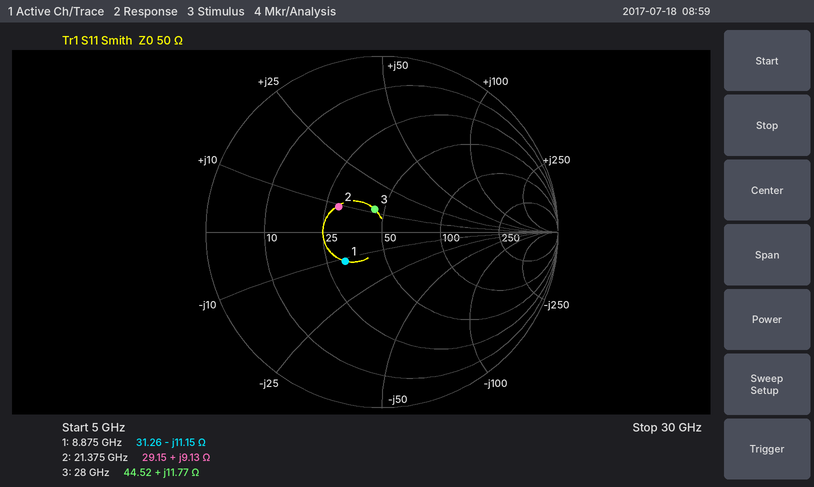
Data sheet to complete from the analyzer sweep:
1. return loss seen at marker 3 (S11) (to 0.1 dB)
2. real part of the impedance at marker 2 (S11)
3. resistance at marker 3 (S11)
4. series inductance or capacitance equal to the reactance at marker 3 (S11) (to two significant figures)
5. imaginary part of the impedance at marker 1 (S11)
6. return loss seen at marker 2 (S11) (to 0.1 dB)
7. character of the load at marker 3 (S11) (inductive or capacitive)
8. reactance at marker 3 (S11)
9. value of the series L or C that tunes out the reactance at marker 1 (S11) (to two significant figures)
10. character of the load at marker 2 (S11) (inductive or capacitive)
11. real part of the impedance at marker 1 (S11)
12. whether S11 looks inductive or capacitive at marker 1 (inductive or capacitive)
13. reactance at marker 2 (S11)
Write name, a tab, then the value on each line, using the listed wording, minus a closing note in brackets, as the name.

return loss seen at marker 3 (S11)	17.3 dB
real part of the impedance at marker 2	29.15 Ω
resistance at marker 3	44.52 Ω
series inductance or capacitance equal to the reactance at marker 3 (S11)	67 pH
imaginary part of the impedance at marker 1	-11.15 Ω
return loss seen at marker 2 (S11)	10.9 dB
character of the load at marker 3 (S11)	inductive
reactance at marker 3	+11.77 Ω
value of the series L or C that tunes out the reactance at marker 1 (S11)	200 pH
character of the load at marker 2 (S11)	inductive
real part of the impedance at marker 1	31.26 Ω
whether S11 looks inductive or capacitive at marker 1	capacitive
reactance at marker 2	+9.13 Ω
